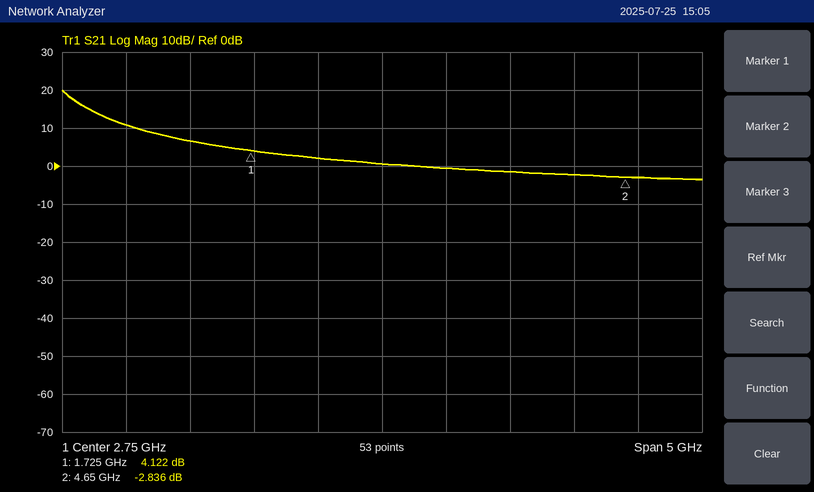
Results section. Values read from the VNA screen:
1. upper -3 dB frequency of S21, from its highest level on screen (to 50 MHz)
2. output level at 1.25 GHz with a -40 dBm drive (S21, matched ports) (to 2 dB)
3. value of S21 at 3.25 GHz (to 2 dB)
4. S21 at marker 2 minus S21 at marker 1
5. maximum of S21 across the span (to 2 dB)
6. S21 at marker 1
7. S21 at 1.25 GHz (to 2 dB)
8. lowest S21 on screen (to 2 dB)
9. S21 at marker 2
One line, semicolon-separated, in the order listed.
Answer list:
350 MHz; -34 dBm; 0 dB; -6.958 dB; 20 dB; 4.122 dB; 6 dB; -4 dB; -2.836 dB
